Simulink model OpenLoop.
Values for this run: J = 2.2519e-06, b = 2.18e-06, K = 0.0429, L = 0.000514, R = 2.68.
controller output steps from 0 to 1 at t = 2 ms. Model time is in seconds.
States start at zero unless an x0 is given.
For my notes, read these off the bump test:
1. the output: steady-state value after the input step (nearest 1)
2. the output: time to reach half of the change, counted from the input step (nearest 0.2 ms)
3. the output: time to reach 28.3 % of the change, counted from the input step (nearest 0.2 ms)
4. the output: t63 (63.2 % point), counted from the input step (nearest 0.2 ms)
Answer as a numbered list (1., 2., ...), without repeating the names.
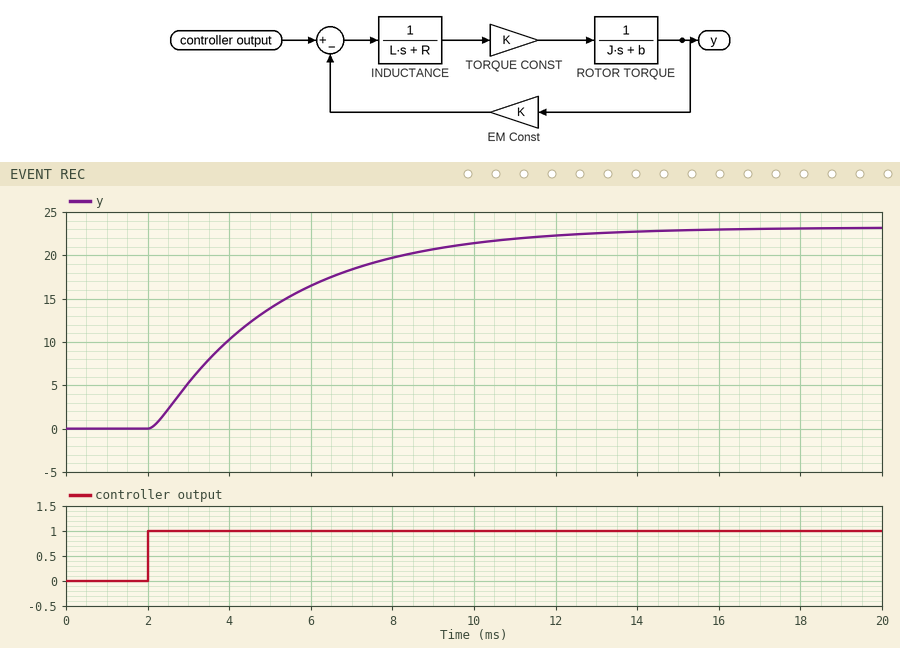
1. 23
2. 2.4 ms
3. 1.2 ms
4. 3.2 ms
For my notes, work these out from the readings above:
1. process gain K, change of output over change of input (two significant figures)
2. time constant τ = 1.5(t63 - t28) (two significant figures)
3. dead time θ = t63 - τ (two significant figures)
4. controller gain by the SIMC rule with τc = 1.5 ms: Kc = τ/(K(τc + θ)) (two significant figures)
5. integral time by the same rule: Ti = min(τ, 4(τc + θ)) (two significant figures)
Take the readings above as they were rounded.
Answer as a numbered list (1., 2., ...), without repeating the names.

1. 23
2. 3.0 ms
3. 0.20 ms
4. 0.077
5. 3.0 ms
